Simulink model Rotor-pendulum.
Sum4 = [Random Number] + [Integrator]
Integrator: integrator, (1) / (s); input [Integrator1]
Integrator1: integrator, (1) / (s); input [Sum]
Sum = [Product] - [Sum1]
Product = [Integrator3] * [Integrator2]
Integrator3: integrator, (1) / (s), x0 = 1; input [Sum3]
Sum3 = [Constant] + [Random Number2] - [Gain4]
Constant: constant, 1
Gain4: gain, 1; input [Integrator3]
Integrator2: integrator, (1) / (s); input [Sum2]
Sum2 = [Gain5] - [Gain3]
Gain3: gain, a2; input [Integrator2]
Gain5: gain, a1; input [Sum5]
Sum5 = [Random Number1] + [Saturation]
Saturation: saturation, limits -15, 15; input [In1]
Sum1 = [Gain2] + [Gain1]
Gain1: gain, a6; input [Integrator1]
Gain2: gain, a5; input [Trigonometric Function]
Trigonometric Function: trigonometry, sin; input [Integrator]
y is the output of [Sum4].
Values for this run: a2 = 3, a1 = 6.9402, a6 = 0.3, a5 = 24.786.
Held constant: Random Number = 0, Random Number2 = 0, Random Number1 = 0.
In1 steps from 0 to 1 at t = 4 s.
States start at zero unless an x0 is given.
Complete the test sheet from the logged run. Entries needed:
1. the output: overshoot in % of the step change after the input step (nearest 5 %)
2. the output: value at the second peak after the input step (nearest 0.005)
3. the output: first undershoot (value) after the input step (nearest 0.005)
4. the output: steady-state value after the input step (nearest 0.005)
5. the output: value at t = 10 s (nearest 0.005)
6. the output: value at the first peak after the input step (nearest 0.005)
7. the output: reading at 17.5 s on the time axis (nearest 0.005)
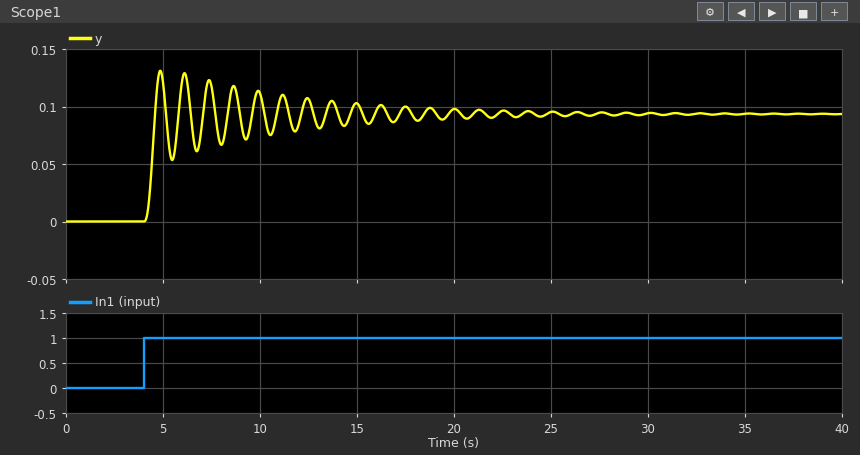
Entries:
40 %
0.130
0.055
0.095
0.110
0.130
0.100
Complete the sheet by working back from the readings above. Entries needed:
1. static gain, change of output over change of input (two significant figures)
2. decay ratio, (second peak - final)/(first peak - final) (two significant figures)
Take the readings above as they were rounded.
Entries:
0.095
1.0
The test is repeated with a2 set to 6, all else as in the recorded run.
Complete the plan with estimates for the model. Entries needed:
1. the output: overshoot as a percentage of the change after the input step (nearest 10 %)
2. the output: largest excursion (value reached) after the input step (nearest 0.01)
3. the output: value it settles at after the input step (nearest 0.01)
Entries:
70 %
0.08
0.05
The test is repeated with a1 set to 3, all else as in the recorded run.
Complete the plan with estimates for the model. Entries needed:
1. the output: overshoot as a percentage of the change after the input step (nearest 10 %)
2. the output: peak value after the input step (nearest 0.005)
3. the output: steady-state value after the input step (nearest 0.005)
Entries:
40 %
0.055
0.040
